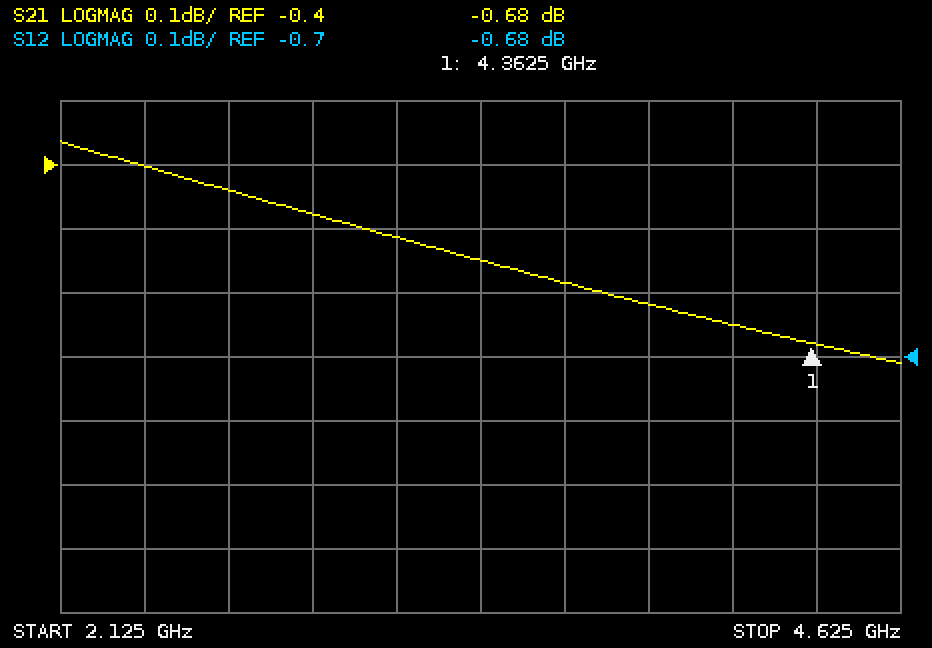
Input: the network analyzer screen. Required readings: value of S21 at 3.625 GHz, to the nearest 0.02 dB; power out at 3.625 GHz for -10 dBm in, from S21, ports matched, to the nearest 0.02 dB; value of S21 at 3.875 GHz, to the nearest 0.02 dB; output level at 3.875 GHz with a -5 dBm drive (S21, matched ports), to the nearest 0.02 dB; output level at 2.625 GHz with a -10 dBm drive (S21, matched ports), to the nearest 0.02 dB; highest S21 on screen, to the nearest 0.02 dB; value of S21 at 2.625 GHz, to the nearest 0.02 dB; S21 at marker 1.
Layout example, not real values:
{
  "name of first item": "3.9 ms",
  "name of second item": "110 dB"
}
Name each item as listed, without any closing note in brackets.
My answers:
{
  "value of S21 at 3.625 GHz, to the nearest 0.02 dB": "-0.58 dB",
  "power out at 3.625 GHz for -10 dBm in, from S21, ports matched, to the nearest 0.02 dB": "-10.58 dBm",
  "value of S21 at 3.875 GHz, to the nearest 0.02 dB": "-0.62 dB",
  "output level at 3.875 GHz with a -5 dBm drive (S21, matched ports), to the nearest 0.02 dB": "-5.62 dBm",
  "output level at 2.625 GHz with a -10 dBm drive (S21, matched ports), to the nearest 0.02 dB": "-10.44 dBm",
  "highest S21 on screen, to the nearest 0.02 dB": "-0.36 dB",
  "value of S21 at 2.625 GHz, to the nearest 0.02 dB": "-0.44 dB",
  "S21 at marker 1": "-0.68 dB"
}
